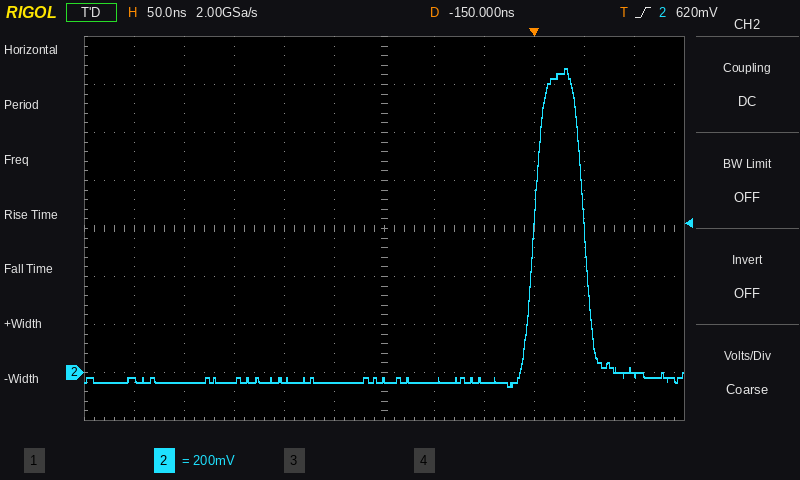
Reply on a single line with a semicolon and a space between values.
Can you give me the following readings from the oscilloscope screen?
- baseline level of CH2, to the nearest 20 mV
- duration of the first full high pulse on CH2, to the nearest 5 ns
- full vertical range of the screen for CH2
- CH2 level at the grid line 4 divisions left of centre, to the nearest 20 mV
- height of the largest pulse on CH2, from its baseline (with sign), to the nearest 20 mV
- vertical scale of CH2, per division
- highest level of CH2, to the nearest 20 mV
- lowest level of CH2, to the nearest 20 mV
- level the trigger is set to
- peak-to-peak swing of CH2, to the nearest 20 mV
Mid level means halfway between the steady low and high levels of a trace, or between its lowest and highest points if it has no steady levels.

-40 mV; 50 ns; 1.6 V; -40 mV; +1.30 V; 200 mV; 1.26 V; -60 mV; 620 mV; 1.32 V
